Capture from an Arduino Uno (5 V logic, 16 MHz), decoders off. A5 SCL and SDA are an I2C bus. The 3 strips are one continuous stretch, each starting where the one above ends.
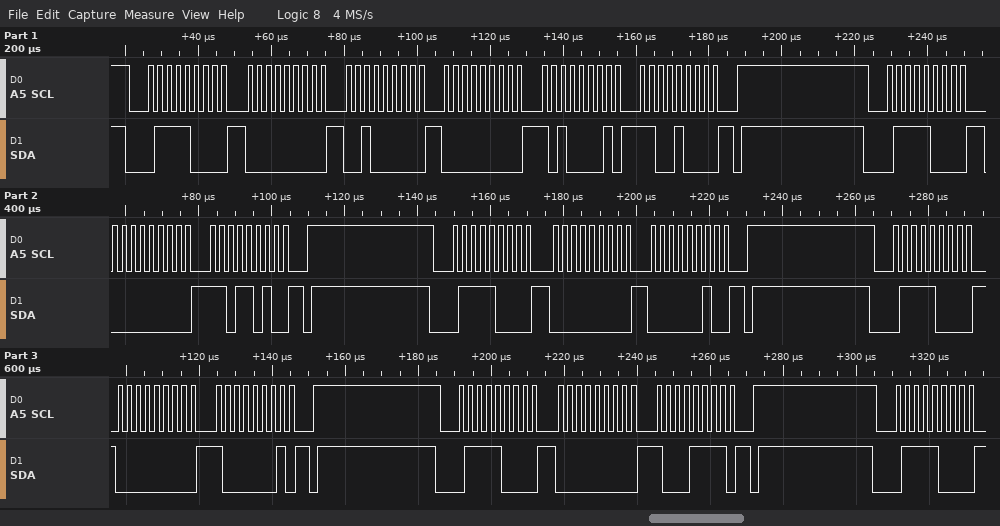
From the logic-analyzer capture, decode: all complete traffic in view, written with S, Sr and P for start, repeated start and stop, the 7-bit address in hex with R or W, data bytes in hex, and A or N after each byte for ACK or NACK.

S 3CW A 00 A 20 A 00 A A1 A C8 A P S 3CW A 00 A DA A P S 3CW A 00 A 02 A P S 3CW A 00 A 81 A P S 3CW A 00 A 8F A P S 3CW A
